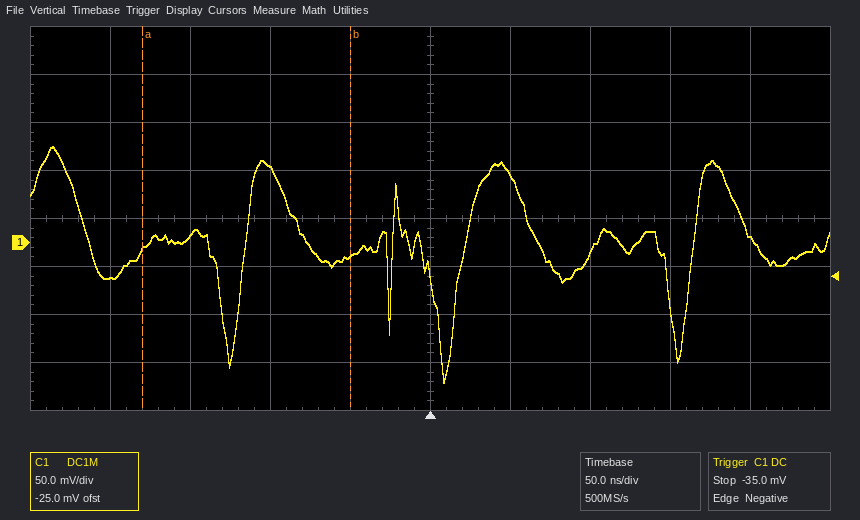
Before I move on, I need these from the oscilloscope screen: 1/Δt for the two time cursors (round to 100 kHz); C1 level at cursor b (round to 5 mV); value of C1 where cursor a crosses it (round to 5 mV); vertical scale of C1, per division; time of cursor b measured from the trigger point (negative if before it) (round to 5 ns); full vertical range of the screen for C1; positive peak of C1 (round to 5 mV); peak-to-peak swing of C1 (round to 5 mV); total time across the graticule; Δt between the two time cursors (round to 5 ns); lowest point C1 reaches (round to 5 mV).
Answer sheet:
7.7 MHz
-15 mV
-10 mV
50 mV
-50 ns
400 mV
100 mV
245 mV
500 ns
130 ns
-145 mV
